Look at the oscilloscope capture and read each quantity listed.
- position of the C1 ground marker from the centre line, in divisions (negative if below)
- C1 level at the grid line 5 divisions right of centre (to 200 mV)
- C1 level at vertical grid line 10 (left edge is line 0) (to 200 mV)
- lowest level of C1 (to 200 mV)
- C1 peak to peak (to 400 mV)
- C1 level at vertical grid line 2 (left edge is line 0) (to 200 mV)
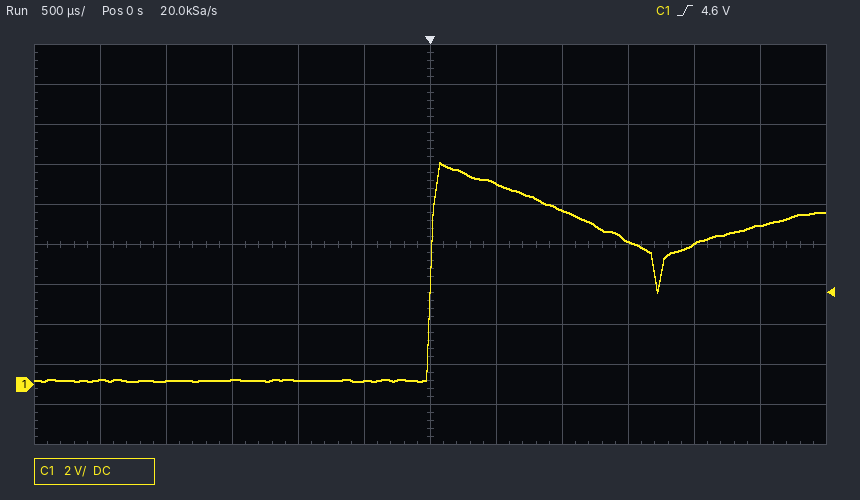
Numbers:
-3.5 div
8.0 V
7.0 V
200 mV
10.8 V
200 mV
